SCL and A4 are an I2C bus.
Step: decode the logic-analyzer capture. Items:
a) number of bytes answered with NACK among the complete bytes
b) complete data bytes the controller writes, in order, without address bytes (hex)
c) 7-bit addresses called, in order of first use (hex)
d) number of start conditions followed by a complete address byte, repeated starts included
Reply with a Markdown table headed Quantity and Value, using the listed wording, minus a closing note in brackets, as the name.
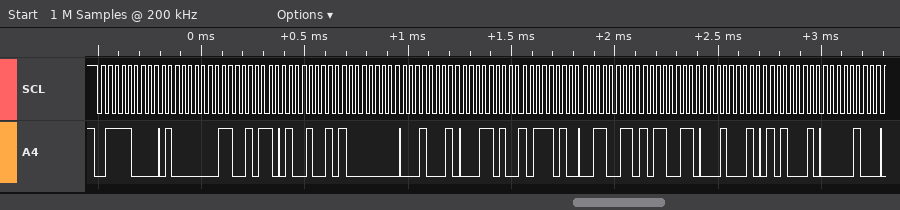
| Quantity | Value |
|---|---|
| number of bytes answered with NACK among the complete bytes | 0 |
| complete data bytes the controller writes, in order, without address bytes | 40 CB 49 80 11 1A BA 33 B3 11 51 04 |
| 7-bit addresses called, in order of first use | 0x3C |
| number of start conditions followed by a complete address byte, repeated starts included | 1 |
